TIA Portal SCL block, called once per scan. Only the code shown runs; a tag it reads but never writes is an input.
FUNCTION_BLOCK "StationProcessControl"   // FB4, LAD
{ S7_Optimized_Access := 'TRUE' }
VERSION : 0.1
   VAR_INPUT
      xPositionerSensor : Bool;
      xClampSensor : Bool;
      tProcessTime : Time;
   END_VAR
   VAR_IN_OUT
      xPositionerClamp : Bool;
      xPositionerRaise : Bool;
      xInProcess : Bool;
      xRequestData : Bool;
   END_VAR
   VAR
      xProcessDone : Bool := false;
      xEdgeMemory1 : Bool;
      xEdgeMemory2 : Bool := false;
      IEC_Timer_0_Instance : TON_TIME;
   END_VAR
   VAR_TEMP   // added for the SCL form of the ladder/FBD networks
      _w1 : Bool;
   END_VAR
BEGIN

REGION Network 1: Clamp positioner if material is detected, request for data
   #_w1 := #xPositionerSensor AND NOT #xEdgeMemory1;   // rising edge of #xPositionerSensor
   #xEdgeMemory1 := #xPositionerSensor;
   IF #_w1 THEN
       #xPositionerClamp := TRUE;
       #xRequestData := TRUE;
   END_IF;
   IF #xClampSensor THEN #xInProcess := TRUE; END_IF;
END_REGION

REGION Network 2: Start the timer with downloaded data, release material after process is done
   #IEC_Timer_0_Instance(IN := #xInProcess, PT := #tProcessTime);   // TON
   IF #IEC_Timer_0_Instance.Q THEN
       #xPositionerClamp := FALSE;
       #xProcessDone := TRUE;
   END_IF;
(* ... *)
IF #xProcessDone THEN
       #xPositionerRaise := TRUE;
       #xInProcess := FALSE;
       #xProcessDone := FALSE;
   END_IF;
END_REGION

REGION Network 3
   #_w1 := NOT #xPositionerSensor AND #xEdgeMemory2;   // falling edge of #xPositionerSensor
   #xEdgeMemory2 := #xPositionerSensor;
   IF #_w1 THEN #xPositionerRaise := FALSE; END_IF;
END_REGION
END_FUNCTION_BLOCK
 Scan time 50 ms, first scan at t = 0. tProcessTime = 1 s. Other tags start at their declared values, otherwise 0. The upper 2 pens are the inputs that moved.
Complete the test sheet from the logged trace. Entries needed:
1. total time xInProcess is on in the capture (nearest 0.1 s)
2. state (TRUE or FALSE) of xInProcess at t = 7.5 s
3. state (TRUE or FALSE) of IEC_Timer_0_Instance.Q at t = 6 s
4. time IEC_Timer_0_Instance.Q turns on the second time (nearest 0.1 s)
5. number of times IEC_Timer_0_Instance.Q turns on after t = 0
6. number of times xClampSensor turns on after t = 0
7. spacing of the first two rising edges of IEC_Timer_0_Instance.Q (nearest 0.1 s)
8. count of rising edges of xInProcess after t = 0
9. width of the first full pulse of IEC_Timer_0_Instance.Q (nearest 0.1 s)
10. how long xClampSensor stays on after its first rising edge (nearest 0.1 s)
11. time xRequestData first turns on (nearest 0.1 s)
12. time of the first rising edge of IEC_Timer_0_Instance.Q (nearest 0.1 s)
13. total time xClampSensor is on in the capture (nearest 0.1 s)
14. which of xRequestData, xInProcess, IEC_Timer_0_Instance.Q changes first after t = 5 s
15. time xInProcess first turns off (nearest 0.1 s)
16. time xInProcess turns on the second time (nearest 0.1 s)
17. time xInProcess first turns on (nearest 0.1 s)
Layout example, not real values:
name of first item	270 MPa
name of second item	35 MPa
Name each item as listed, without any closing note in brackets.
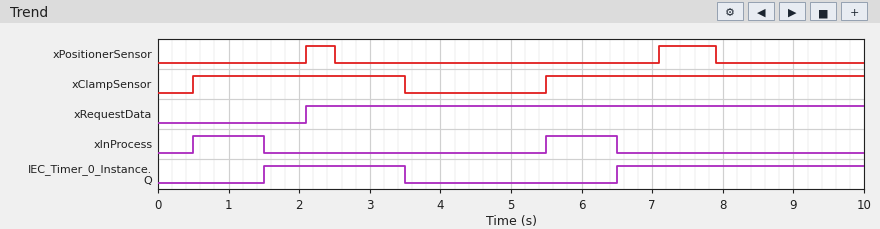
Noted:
total time xInProcess is on in the capture	2.0 s
state (TRUE or FALSE) of xInProcess at t = 7.5 s	FALSE
state (TRUE or FALSE) of IEC_Timer_0_Instance.Q at t = 6 s	FALSE
time IEC_Timer_0_Instance.Q turns on the second time	6.5 s
number of times IEC_Timer_0_Instance.Q turns on after t = 0	2
number of times xClampSensor turns on after t = 0	2
spacing of the first two rising edges of IEC_Timer_0_Instance.Q	5.0 s
count of rising edges of xInProcess after t = 0	2
width of the first full pulse of IEC_Timer_0_Instance.Q	2.0 s
how long xClampSensor stays on after its first rising edge	3.0 s
time xRequestData first turns on	2.1 s
time of the first rising edge of IEC_Timer_0_Instance.Q	1.5 s
total time xClampSensor is on in the capture	7.5 s
which of xRequestData, xInProcess, IEC_Timer_0_Instance.Q changes first after t = 5 s	xInProcess
time xInProcess first turns off	1.5 s
time xInProcess turns on the second time	5.5 s
time xInProcess first turns on	0.5 s
